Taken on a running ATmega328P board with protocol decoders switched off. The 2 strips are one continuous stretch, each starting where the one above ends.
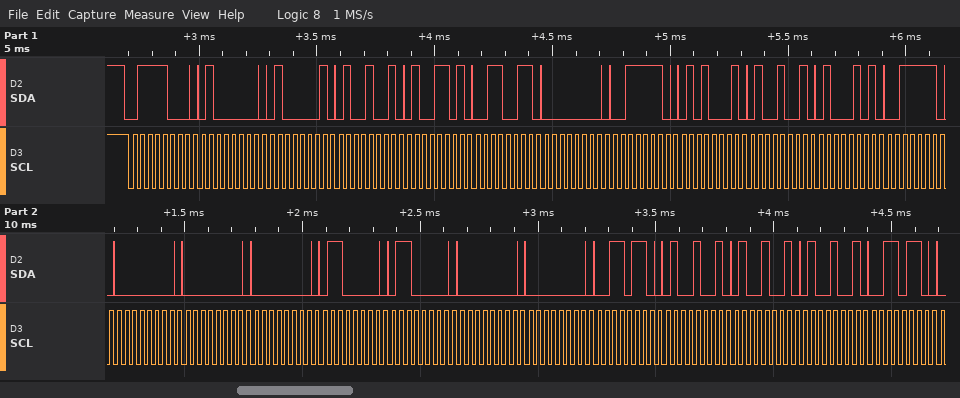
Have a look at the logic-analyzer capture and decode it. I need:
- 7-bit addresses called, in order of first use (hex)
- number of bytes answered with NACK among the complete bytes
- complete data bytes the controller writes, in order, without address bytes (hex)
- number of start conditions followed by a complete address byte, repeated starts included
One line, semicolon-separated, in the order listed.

0x3C; 0; 40 41 49 4D 33 00 3E 51 49 45 3E 00 00 00 60 60 00 00 36 49 49 49 36; 1
